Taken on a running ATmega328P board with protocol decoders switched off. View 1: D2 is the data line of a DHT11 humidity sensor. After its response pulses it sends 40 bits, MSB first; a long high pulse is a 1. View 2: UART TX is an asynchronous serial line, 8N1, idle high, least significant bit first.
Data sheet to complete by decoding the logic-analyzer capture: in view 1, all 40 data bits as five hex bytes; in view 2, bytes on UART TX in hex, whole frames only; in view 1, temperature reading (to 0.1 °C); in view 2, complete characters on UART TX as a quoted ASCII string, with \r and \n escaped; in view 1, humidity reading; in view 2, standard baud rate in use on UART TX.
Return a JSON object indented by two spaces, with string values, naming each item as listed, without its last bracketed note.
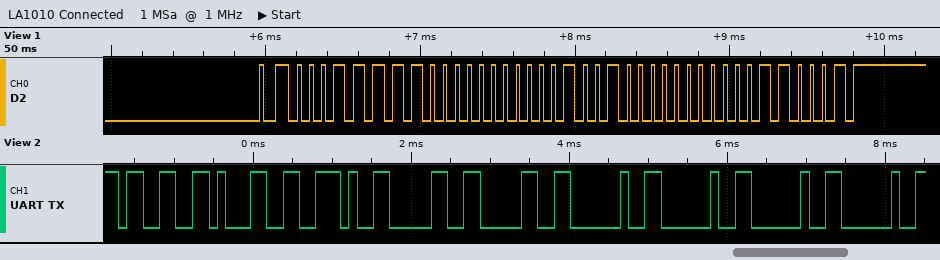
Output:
{
  "in view 1, all 40 data bits as five hex bytes": "1F 00 12 00 31",
  "in view 2, bytes on UART TX in hex, whole frames only": "0x33 0x31 0x2E 0x30 0x30 0x20 0x20 0x20 0x20",
  "in view 1, temperature reading": "18.0 °C",
  "in view 2, complete characters on UART TX as a quoted ASCII string, with \\r and \\n escaped": "\"31.00    \"",
  "in view 1, humidity reading": "31 %",
  "in view 2, standard baud rate in use on UART TX": "9600 baud"
}
